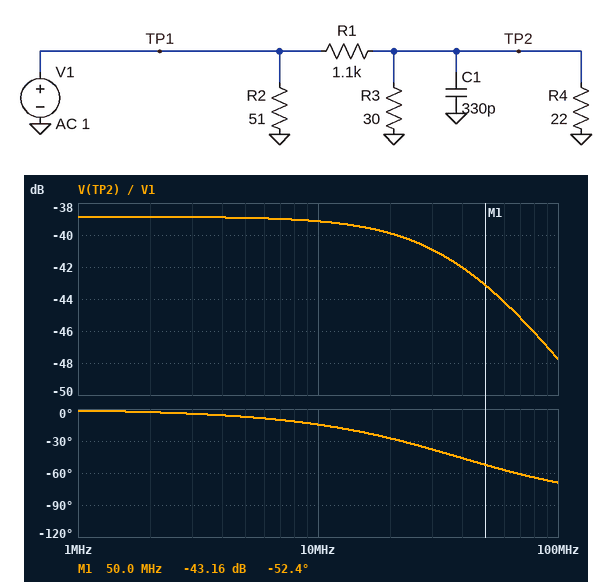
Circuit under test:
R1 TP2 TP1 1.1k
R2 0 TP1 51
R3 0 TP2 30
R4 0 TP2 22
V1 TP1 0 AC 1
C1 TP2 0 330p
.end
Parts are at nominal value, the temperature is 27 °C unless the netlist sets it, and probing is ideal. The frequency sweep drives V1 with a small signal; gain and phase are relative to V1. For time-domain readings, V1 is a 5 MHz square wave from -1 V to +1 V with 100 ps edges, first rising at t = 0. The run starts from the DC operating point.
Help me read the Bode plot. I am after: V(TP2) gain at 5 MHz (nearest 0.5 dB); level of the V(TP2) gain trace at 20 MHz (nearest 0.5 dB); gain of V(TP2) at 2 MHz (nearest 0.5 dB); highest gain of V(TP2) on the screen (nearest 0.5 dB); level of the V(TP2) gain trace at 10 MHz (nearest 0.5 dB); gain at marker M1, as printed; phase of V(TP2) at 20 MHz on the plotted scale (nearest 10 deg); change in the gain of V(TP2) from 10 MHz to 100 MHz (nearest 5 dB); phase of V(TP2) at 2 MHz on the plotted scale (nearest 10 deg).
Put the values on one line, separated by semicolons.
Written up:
-39.0 dB; -40.0 dB; -39.0 dB; -39.0 dB; -39.0 dB; -43.16 dB; -30 deg; -10 dB; 0 deg
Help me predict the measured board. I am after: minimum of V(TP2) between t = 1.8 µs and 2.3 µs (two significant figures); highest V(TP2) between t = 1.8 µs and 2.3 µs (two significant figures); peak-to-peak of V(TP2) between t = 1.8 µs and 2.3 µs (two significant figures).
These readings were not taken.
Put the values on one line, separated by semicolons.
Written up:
-11 mV; 11 mV; 23 mV
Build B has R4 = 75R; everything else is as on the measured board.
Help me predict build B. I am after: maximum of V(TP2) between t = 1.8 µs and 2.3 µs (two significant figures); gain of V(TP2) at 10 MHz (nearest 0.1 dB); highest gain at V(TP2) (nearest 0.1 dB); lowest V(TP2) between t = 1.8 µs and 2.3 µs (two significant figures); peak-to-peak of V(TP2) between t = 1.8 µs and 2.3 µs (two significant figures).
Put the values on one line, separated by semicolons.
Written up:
19 mV; -35.1 dB; -34.4 dB; -19 mV; 38 mV
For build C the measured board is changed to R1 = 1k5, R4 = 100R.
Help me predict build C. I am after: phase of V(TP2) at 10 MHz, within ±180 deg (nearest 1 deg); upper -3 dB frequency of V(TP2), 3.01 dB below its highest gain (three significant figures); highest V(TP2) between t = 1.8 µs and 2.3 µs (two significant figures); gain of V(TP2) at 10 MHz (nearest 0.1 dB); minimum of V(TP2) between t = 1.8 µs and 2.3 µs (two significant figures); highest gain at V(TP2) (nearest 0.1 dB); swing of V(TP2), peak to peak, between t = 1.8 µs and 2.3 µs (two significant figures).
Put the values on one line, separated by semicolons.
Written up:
-25 deg; 21.2 MHz; 15 mV; -37.3 dB; -15 mV; -36.4 dB; 30 mV
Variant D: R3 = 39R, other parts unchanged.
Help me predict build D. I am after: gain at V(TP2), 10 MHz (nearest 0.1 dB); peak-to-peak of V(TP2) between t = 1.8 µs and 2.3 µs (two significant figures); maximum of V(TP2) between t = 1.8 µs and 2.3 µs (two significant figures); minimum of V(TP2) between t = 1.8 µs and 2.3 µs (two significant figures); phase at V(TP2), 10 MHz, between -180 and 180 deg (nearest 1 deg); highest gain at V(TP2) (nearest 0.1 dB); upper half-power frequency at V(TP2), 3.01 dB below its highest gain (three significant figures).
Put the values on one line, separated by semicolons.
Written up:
-38.3 dB; 25 mV; 13 mV; -13 mV; -16 deg; -38.0 dB; 34.7 MHz
